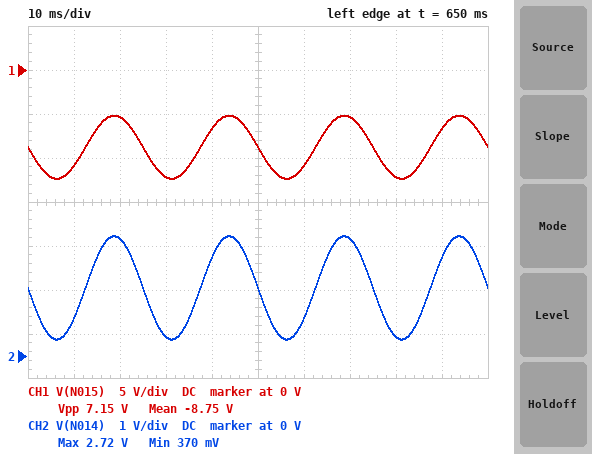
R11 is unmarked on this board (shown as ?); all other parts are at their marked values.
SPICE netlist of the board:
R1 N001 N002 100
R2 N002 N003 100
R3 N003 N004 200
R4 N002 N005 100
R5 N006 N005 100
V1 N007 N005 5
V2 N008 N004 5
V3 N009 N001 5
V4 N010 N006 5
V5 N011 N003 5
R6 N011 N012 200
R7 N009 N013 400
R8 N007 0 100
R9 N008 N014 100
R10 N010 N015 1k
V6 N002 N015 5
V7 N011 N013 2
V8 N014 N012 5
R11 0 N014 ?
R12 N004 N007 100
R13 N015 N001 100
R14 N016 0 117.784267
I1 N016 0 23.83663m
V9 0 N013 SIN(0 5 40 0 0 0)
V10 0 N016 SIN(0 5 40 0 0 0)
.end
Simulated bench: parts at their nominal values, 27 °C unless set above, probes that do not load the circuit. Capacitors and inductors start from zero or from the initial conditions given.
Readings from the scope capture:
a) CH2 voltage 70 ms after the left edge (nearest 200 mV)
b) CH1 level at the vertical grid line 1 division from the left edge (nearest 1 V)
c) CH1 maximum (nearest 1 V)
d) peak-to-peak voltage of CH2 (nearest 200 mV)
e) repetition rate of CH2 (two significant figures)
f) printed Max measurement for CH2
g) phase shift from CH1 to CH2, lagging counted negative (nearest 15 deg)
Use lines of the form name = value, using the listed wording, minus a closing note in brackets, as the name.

CH2 voltage 70 ms after the left edge = 2.6 V
CH1 level at the vertical grid line 1 division from the left edge = -11 V
CH1 maximum = -5 V
peak-to-peak voltage of CH2 = 2.4 V
repetition rate of CH2 = 40 Hz
printed Max measurement for CH2 = 2.72 V
phase shift from CH1 to CH2, lagging counted negative = 0 deg
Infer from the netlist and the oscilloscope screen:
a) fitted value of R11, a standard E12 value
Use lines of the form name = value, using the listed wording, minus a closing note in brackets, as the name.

fitted value of R11, a standard E12 value = 39 Ω
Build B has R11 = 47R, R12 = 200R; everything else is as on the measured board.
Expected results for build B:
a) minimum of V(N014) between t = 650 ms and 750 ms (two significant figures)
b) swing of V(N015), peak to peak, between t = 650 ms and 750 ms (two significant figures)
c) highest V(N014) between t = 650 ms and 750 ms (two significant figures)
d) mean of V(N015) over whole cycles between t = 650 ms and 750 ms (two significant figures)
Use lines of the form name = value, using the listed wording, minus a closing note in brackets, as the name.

minimum of V(N014) between t = 650 ms and 750 ms = 300 mV
swing of V(N015), peak to peak, between t = 650 ms and 750 ms = 7.1 V
highest V(N014) between t = 650 ms and 750 ms = 3.0 V
mean of V(N015) over whole cycles between t = 650 ms and 750 ms = -8.6 V
